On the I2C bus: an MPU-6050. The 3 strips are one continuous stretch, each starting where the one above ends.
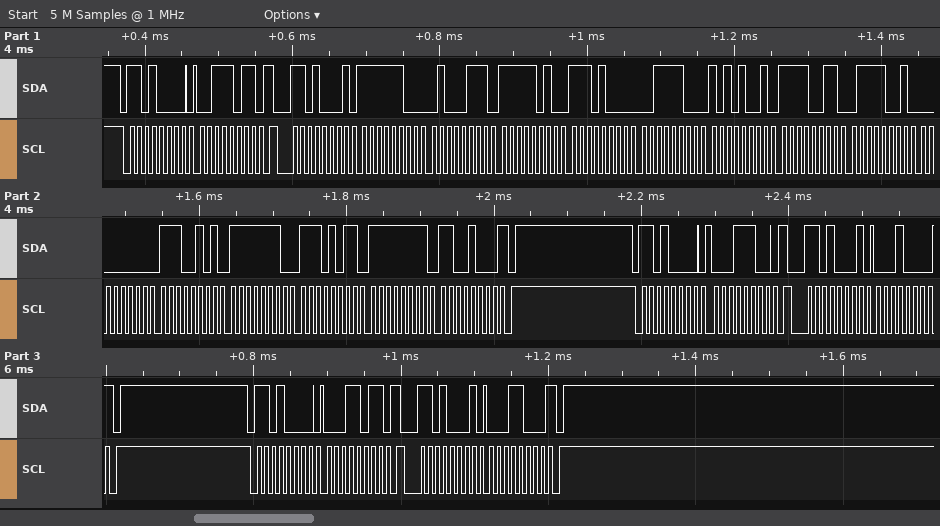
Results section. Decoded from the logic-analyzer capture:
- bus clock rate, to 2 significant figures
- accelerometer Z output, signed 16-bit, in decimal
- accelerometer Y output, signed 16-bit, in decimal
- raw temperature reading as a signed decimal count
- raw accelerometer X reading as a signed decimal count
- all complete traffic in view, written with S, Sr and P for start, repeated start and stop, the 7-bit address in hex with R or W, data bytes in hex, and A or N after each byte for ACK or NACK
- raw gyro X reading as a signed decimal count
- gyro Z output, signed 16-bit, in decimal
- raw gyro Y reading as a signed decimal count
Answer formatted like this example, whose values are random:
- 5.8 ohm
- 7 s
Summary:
- 100 kHz
- 15529
- -1304
- -3207
- -953
- S 68W A 3B A Sr 68R A FC A 47 A FA A E8 A 3C A A9 A F3 A 79 A 00 A E5 A FE A EB A FF A C8 N P S 68W A 1C A Sr 68R A 10 N P S 68W A 1B A Sr 68R A 18 N P
- 229
- -56
- -277
